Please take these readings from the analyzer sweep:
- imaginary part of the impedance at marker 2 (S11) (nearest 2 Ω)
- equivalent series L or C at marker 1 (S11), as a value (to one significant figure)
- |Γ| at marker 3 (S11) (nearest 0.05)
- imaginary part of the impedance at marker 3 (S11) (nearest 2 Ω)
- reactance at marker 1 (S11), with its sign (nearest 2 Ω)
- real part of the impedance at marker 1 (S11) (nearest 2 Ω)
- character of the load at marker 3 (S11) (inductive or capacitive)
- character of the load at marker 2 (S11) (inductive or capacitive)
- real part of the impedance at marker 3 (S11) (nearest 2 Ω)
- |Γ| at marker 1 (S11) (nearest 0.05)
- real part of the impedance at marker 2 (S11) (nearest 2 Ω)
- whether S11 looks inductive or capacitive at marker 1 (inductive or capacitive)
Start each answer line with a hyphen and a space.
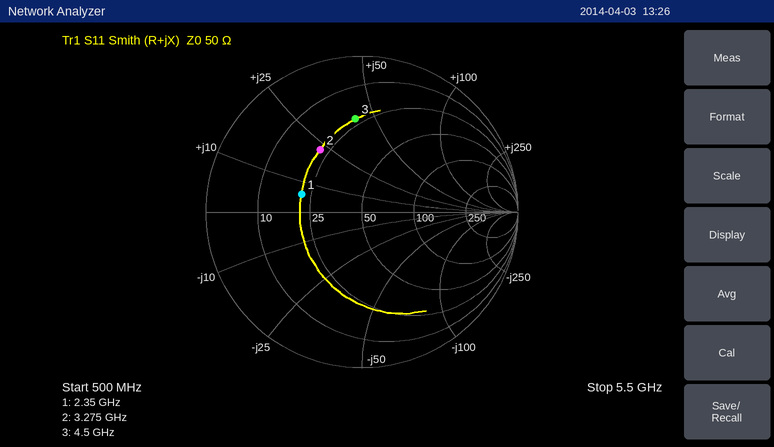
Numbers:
- +22 Ω
- 400 pH
- 0.60
- +42 Ω
- +6 Ω
- 22 Ω
- inductive
- inductive
- 22 Ω
- 0.40
- 22 Ω
- inductive
